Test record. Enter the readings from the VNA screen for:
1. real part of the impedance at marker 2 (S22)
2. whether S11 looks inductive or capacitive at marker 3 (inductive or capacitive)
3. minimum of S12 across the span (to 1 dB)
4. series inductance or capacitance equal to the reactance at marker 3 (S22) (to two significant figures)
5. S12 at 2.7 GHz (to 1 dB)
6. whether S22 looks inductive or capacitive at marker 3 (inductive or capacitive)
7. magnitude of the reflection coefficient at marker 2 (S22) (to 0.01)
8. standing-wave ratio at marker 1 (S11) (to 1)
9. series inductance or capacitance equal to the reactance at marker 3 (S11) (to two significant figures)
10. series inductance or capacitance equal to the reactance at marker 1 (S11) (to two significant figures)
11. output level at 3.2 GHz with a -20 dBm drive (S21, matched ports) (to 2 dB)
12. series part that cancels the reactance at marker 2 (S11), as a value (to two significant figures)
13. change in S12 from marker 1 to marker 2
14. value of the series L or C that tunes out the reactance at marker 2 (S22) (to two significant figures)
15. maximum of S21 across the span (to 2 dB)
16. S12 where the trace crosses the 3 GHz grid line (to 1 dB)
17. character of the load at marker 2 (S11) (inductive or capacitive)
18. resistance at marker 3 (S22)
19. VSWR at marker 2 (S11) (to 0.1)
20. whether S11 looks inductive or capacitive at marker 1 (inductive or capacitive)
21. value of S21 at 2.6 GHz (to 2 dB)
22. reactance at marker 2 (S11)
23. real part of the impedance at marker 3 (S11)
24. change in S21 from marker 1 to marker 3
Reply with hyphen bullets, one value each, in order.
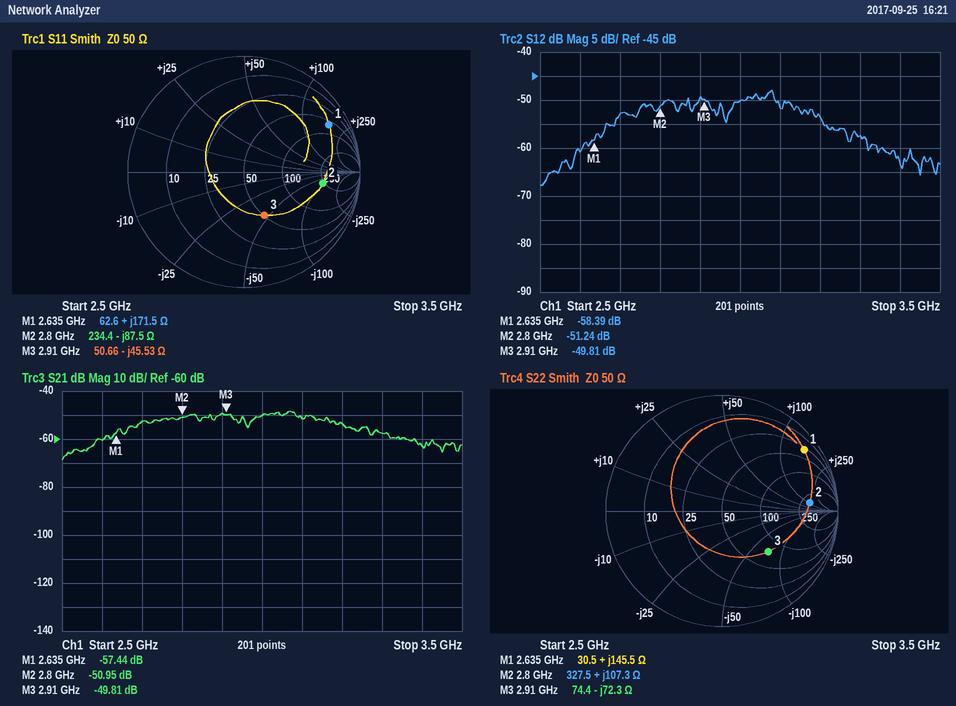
- 327.5 Ω
- capacitive
- -68 dB
- 760 fF
- -53 dB
- capacitive
- 0.76
- 11
- 1.2 pF
- 10 nH
- -74 dBm
- 5.0 nH
- 7.15 dB
- 530 fF
- -48 dB
- -50 dB
- capacitive
- 74.4 Ω
- 5.4
- inductive
- -60 dB
- -87.5 Ω
- 50.66 Ω
- 7.63 dB
